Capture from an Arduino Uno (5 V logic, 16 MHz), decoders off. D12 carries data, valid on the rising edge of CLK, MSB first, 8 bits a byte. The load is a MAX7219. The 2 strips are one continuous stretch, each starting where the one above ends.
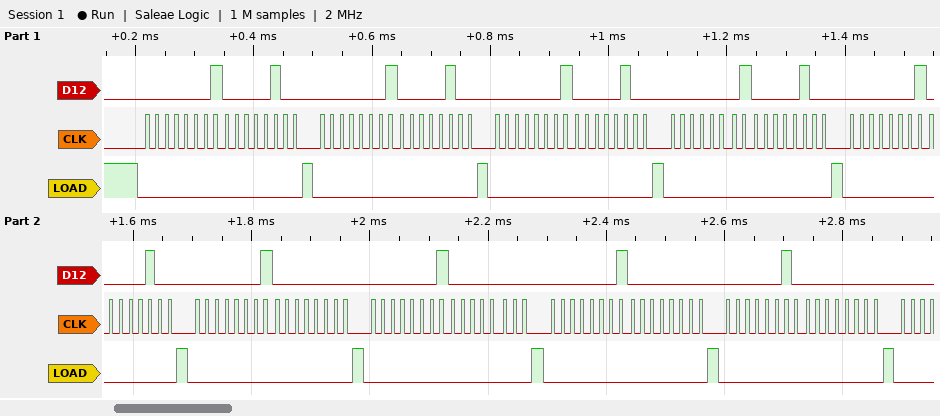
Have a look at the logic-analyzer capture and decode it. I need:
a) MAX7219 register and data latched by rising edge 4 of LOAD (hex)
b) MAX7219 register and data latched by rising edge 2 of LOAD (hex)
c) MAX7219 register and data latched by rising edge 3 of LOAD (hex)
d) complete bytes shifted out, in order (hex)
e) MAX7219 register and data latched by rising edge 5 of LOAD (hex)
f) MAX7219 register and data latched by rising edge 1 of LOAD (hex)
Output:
register 0x1, data 0x04
register 0x1, data 0x04
register 0x1, data 0x04
01 04 01 04 01 04 01 04 01 04 01 00 01 00 01 00 02 00
register 0x1, data 0x04
register 0x1, data 0x04
